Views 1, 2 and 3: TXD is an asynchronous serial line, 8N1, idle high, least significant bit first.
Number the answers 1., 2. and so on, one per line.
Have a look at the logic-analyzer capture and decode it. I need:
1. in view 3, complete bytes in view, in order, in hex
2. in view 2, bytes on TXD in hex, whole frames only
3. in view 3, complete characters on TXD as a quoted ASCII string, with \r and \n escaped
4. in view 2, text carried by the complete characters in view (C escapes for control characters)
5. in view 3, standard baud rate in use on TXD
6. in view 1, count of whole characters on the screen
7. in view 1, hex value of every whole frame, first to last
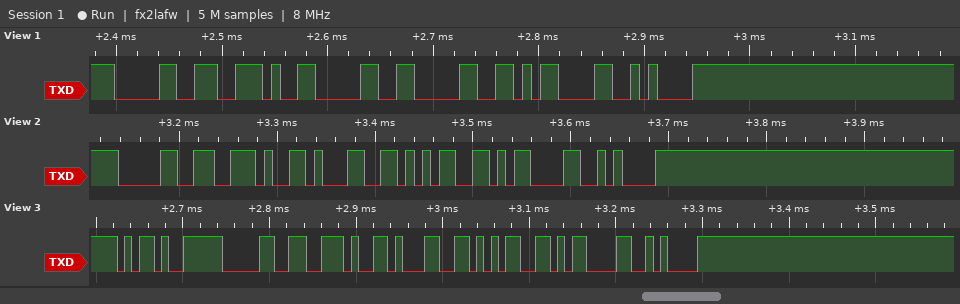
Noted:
1. 0x2D 0x30 0x2E 0x31 0x35 0x0D 0x0A
2. 30 2E 31 35 0D 0A
3. "-0.15\r\n"
4. "0.15\r\n"
5. 115200 baud
6. 6
7. 30 2E 30 30 0D 0A
